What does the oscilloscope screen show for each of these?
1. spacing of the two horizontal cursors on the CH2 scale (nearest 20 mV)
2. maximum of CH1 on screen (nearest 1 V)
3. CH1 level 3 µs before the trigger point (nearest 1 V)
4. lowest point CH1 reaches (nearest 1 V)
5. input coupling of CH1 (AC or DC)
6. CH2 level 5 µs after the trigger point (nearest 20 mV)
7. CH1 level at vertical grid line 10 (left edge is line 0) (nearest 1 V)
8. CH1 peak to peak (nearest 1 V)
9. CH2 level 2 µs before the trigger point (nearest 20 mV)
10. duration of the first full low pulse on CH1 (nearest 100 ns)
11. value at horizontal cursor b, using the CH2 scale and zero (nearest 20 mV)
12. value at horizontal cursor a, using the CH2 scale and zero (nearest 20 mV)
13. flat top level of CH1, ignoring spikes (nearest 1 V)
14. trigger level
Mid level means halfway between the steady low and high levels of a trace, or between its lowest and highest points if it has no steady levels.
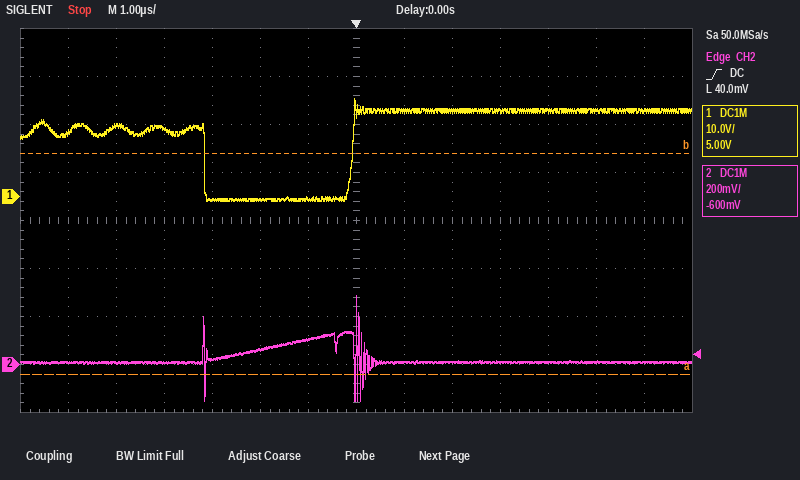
920 mV
20 V
-1 V
-1 V
DC
20 mV
18 V
21 V
60 mV
3.1 µs
880 mV
-40 mV
18 V
40.0 mV
